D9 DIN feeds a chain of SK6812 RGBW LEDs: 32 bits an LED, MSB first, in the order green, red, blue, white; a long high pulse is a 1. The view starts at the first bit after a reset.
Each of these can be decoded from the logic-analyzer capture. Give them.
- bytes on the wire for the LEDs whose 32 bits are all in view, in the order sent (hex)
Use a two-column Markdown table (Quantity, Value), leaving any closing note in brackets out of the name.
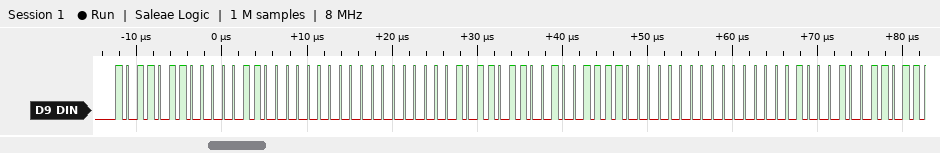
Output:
| Quantity | Value |
|---|---|
| bytes on the wire for the LEDs whose 32 bits are all in view, in the order sent | B6 0C 00 00 B6 4F 00 00 |
